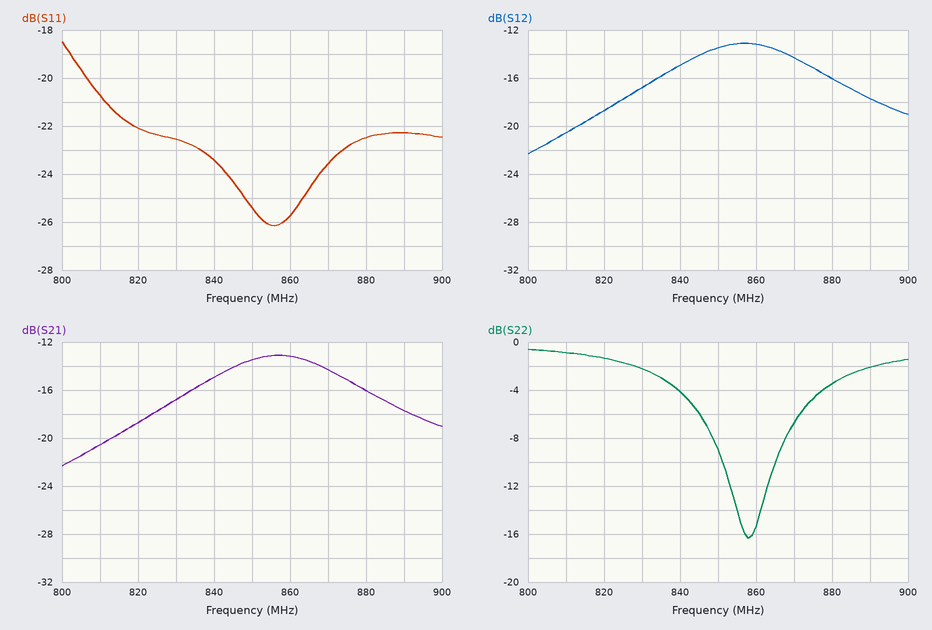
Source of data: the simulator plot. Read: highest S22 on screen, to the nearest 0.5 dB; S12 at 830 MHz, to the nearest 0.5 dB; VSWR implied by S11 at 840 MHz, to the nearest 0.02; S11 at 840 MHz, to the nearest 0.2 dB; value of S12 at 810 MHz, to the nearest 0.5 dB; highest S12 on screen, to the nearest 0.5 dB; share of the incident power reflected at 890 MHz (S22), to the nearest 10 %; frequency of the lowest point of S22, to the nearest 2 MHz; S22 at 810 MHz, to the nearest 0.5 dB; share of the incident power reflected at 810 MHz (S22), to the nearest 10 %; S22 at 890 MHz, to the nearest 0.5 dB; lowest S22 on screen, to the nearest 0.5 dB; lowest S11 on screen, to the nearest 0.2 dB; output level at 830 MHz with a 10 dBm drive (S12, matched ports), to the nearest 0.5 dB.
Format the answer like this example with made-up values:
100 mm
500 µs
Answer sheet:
-0.5 dB
-17.0 dB
1.14
-23.4 dB
-20.5 dB
-13.0 dB
60 %
858 MHz
-1.0 dB
80 %
-2.0 dB
-16.5 dB
-26.2 dB
-7.0 dBm
